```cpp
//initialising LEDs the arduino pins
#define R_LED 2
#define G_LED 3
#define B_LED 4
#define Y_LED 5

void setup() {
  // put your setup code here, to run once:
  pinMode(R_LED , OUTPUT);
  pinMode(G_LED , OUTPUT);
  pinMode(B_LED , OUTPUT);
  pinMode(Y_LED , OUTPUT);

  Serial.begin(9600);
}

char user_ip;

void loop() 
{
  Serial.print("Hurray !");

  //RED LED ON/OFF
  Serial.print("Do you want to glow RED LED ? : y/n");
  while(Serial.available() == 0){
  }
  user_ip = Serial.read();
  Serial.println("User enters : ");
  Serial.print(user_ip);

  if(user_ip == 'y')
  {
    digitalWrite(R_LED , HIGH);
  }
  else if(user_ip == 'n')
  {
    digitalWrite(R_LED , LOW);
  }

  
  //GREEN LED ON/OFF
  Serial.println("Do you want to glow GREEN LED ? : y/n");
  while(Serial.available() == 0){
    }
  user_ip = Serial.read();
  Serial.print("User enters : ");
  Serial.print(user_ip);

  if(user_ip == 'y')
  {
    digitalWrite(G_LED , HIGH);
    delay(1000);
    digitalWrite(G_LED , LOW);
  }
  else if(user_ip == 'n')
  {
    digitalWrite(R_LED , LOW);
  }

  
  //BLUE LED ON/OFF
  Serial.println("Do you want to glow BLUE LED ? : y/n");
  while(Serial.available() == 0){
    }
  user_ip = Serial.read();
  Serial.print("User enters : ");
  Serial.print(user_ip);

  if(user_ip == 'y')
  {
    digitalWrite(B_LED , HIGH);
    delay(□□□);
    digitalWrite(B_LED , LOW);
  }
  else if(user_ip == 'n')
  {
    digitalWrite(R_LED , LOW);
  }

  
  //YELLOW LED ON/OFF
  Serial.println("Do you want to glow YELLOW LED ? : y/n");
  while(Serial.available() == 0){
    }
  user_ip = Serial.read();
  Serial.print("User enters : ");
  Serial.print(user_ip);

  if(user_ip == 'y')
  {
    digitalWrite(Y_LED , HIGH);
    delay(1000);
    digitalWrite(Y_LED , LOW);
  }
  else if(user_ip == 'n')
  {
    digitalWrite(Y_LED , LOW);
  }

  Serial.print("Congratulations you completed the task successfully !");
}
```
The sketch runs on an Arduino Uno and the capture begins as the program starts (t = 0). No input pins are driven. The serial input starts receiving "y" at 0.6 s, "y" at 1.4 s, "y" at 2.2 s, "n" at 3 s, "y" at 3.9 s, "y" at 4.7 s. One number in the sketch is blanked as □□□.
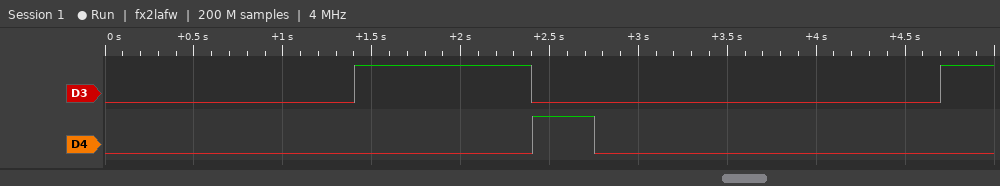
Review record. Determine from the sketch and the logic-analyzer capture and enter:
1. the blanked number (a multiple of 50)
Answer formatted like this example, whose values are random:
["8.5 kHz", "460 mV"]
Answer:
["350"]
